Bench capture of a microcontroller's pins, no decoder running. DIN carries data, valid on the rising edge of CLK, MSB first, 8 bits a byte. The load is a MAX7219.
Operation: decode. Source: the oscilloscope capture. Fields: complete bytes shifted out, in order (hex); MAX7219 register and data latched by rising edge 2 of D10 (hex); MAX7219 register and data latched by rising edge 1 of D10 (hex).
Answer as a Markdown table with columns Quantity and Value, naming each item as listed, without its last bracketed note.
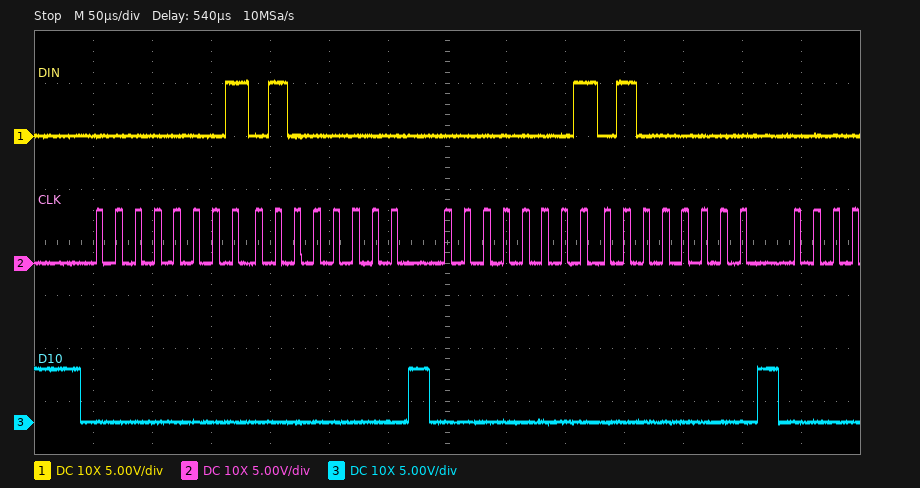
| Quantity | Value |
|---|---|
| complete bytes shifted out, in order | 01 40 01 40 |
| MAX7219 register and data latched by rising edge 2 of D10 | register 0x1, data 0x40 |
| MAX7219 register and data latched by rising edge 1 of D10 | register 0x1, data 0x40 |
